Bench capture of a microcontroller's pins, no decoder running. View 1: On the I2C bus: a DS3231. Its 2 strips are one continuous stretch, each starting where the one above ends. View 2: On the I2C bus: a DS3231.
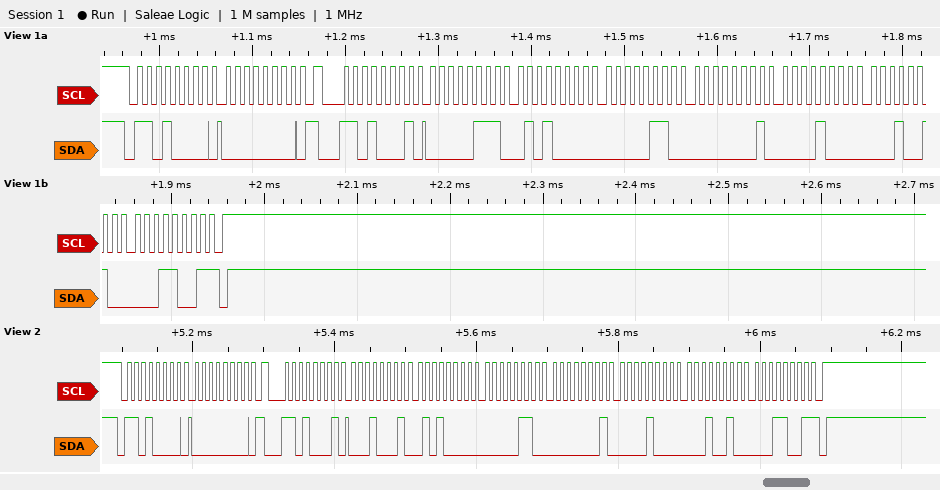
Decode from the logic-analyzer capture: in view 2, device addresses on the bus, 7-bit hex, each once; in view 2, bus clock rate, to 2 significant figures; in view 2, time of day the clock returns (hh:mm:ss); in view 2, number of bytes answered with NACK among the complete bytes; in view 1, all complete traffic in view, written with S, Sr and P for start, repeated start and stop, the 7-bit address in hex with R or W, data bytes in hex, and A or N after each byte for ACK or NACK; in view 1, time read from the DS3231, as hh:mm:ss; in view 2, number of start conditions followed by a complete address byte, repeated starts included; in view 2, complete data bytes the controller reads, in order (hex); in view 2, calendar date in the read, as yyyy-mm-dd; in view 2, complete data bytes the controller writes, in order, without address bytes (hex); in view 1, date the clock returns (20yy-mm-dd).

0x68
100 kHz
06:50:11
1
S 68W A 00 A Sr 68R A 07 A 50 A 06 A 01 A 08 A 12 A 19 N P
06:50:07
2
11 50 06 01 08 12 19
2019-12-08
00
2019-12-08
